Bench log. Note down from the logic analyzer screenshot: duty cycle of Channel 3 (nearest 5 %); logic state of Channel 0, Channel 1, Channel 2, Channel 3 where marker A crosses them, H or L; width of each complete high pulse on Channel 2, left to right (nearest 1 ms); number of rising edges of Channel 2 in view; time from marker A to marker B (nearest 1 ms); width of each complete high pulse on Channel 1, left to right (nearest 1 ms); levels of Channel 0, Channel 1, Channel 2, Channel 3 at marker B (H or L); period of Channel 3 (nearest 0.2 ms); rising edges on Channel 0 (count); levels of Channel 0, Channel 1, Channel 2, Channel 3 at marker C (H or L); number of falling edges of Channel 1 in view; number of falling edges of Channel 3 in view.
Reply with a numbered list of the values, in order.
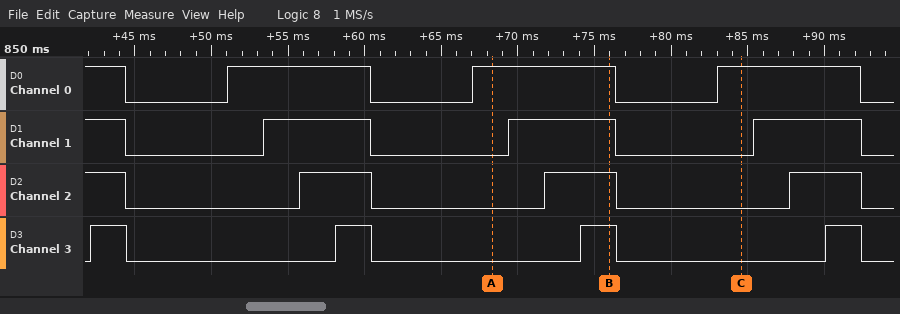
1. 15 %
2. Channel 0=H, Channel 1=L, Channel 2=L, Channel 3=L
3. 5 ms, 5 ms, 5 ms
4. 3
5. 8 ms
6. 7 ms, 7 ms, 7 ms
7. Channel 0=H, Channel 1=H, Channel 2=H, Channel 3=H
8. 16 ms
9. 3
10. Channel 0=H, Channel 1=L, Channel 2=L, Channel 3=L
11. 4
12. 4
